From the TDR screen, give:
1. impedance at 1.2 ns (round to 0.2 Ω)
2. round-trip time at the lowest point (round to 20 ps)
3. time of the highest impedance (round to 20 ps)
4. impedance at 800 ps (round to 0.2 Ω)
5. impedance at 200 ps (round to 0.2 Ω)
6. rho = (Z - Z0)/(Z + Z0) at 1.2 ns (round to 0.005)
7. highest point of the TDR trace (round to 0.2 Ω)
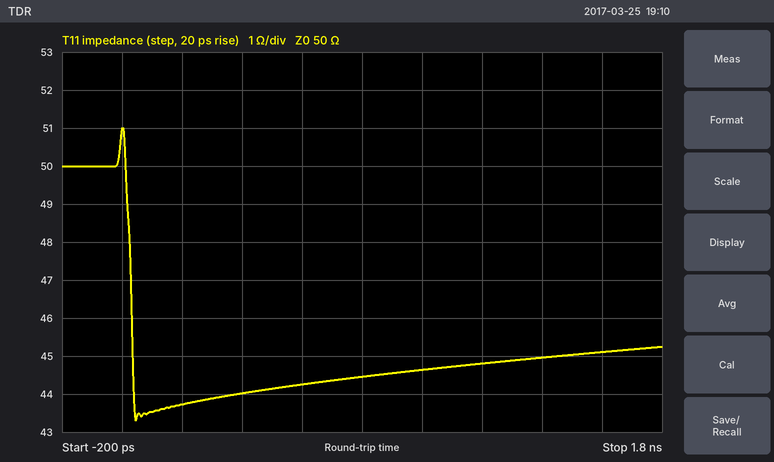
44.8 Ω
40 ps
0 ps
44.4 Ω
43.8 Ω
-0.055
51.0 Ω
